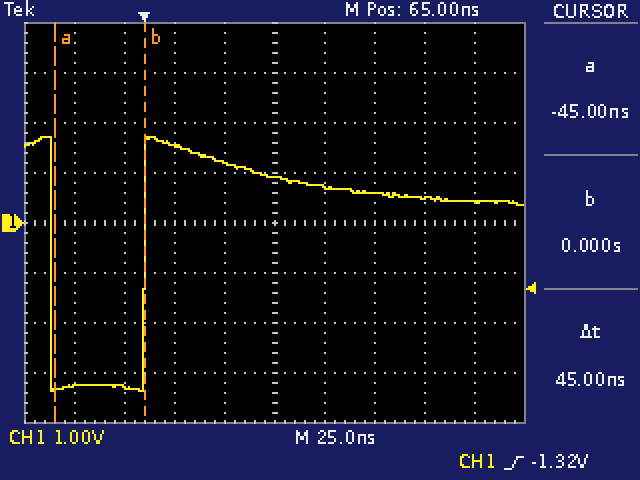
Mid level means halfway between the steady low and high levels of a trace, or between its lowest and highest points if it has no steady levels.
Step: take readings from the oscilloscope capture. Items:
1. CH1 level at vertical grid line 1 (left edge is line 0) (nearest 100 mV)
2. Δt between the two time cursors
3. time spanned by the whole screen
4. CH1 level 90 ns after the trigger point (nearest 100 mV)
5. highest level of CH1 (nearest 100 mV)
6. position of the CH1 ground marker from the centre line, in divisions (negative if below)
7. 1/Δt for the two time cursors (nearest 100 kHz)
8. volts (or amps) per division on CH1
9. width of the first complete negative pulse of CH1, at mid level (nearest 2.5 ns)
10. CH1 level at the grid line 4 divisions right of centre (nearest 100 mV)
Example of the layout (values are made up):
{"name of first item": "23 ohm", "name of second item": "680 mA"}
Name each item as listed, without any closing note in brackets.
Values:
{"CH1 level at vertical grid line 1 (left edge is line 0)": "-3.3 V", "Δt between the two time cursors": "45 ns", "time spanned by the whole screen": "250 ns", "CH1 level 90 ns after the trigger point": "700 mV", "highest level of CH1": "1.7 V", "position of the CH1 ground marker from the centre line, in divisions": "0.0 div", "1/Δt for the two time cursors": "22.2 MHz", "volts (or amps) per division on CH1": "1 V", "width of the first complete negative pulse of CH1, at mid level": "47.5 ns", "CH1 level at the grid line 4 divisions right of centre": "400 mV"}
